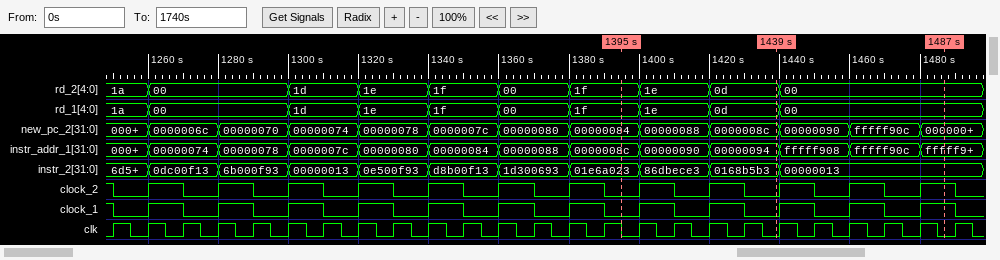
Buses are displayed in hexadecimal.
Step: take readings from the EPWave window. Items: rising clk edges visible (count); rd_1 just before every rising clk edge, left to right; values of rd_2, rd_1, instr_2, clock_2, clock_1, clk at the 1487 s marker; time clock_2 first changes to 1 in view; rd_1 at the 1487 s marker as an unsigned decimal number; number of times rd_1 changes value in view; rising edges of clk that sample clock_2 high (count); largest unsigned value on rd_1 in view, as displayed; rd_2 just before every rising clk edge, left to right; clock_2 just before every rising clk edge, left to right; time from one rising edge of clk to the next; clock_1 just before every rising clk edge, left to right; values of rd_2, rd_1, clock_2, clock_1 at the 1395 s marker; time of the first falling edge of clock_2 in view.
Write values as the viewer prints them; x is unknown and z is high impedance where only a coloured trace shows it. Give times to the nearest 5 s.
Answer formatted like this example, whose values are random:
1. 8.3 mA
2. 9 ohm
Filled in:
1. 25
2. 1a, 1a, 00, 00, 00, 00, 1d, 1d, 1e, 1e, 1f, 1f, 00, 00, 1f, 1f, 1e, 1e, 0d, 0d, 00, 00, 00, 00, 00
3. rd_2=00, rd_1=00, instr_2=00000013, clock_2=1, clock_1=1, clk=0
4. 1260 s
5. 0
6. 9
7. 13
8. 1f
9. 1a, 1a, 00, 00, 00, 00, 1d, 1d, 1e, 1e, 1f, 1f, 00, 00, 1f, 1f, 1e, 1e, 0d, 0d, 00, 00, 00, 00, 00
10. 1 0 1 0 1 0 1 0 1 0 1 0 1 0 1 0 1 0 1 0 1 0 1 0 1
11. 10 s
12. 1 0 1 0 1 0 1 0 1 0 1 0 1 0 1 0 1 0 1 0 1 0 1 0 1
13. rd_2=1f, rd_1=1f, clock_2=0, clock_1=0
14. 1250 s
